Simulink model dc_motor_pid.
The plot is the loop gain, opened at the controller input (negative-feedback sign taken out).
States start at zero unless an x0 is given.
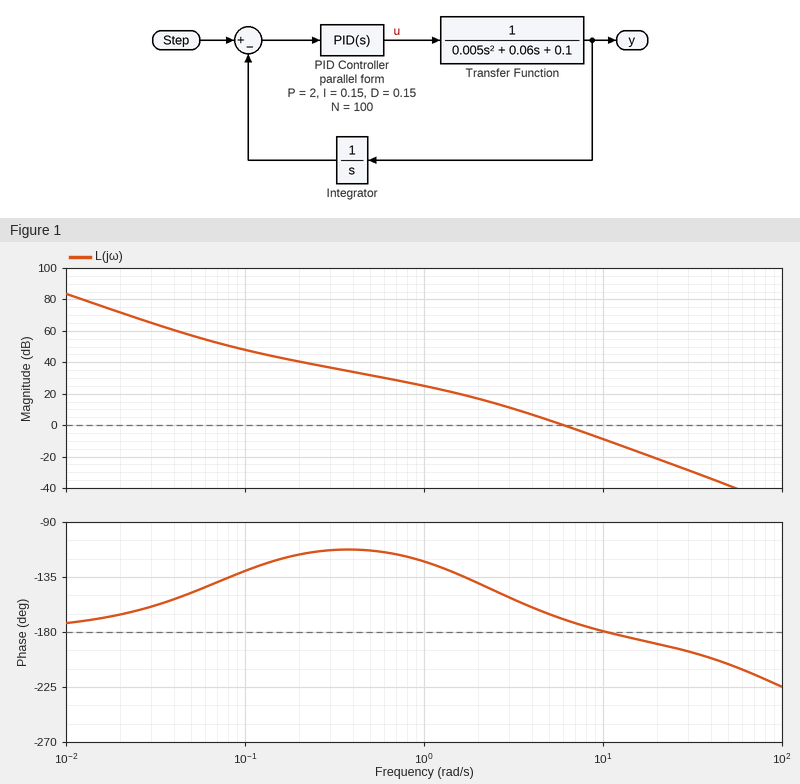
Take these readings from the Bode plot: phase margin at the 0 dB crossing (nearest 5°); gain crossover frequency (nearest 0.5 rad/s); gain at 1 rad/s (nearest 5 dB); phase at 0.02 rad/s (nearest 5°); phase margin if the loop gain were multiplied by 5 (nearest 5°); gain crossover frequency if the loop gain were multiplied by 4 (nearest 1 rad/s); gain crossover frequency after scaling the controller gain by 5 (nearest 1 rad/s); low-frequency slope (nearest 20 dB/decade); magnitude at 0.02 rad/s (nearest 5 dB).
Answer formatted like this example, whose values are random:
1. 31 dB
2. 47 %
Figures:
1. 10°
2. 6.0 rad/s
3. 25 dB
4. -165°
5. -5°
6. 12 rad/s
7. 13 rad/s
8. -40 dB/decade
9. 70 dB
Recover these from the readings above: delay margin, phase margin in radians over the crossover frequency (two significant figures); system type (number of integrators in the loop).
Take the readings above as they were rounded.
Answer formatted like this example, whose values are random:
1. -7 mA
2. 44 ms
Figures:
1. 0.029 s
2. 2
